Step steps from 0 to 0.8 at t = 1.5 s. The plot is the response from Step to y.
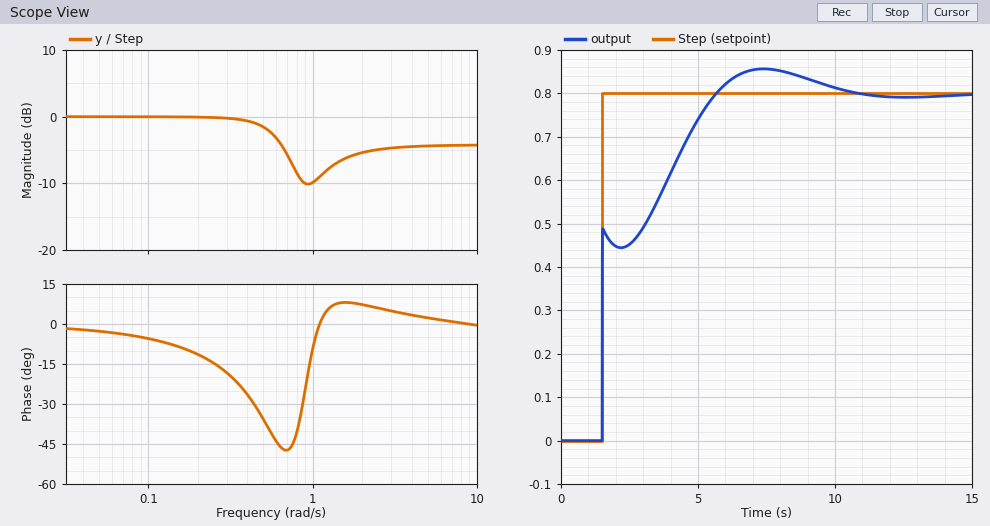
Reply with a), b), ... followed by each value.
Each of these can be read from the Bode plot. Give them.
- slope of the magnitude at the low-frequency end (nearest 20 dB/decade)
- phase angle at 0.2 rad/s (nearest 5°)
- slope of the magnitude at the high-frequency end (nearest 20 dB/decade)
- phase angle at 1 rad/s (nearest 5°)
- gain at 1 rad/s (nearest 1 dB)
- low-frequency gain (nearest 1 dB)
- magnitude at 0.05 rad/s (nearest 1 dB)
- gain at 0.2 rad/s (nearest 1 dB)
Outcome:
a) 0 dB/decade
b) -10°
c) 0 dB/decade
d) -10°
e) -10 dB
f) 0 dB
g) 0 dB
h) 0 dB
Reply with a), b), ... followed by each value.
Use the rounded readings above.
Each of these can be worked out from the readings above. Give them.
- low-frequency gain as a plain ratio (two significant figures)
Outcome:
a) 1.0
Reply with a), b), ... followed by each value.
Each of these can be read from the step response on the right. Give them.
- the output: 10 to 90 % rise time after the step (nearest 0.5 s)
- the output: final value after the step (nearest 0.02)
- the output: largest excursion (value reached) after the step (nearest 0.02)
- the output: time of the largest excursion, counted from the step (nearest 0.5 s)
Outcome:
a) 3.5 s
b) 0.80
c) 0.86
d) 6.0 s
